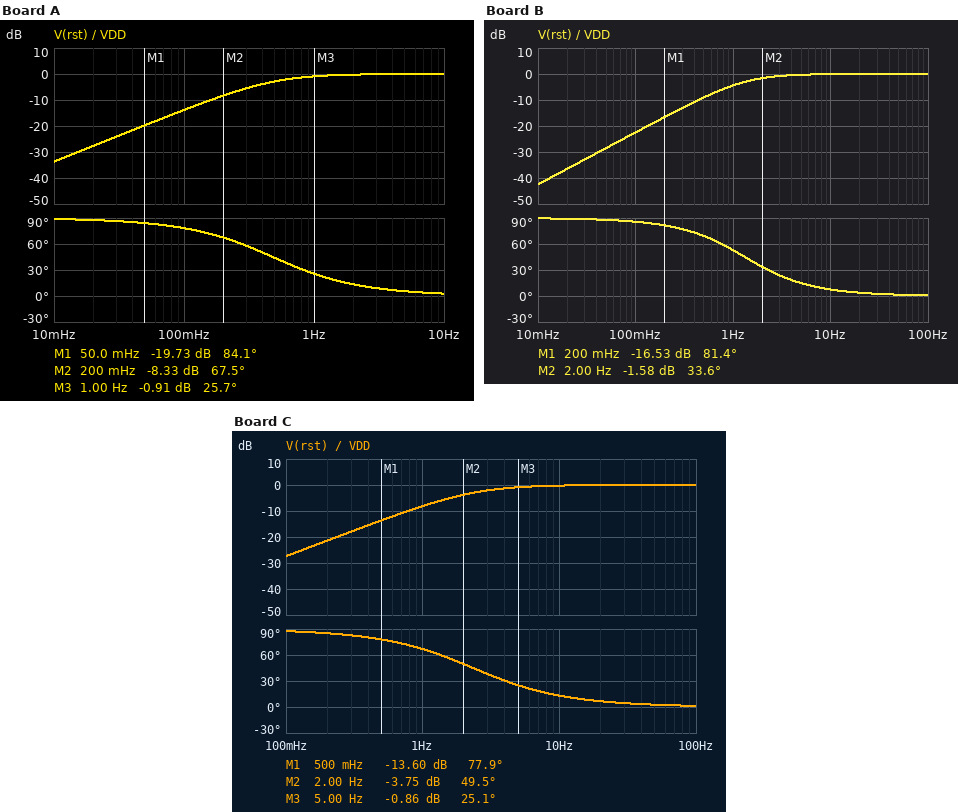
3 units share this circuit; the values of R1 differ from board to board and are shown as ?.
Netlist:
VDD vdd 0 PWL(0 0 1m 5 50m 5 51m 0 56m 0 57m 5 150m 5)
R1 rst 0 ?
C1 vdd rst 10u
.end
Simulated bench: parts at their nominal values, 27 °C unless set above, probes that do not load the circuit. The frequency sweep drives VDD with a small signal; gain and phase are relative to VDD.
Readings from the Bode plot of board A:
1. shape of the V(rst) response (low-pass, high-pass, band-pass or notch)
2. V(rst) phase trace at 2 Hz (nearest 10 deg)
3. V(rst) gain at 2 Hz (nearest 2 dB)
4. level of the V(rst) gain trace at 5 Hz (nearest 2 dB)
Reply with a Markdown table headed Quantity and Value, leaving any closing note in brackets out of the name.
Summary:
| Quantity | Value |
|---|---|
| shape of the V(rst) response | high-pass |
| V(rst) phase trace at 2 Hz | 10 deg |
| V(rst) gain at 2 Hz | 0 dB |
| level of the V(rst) gain trace at 5 Hz | 0 dB |
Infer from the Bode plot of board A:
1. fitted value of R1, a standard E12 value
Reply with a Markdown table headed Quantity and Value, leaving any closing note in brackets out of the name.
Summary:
| Quantity | Value |
|---|---|
| fitted value of R1, a standard E12 value | 33 kΩ |
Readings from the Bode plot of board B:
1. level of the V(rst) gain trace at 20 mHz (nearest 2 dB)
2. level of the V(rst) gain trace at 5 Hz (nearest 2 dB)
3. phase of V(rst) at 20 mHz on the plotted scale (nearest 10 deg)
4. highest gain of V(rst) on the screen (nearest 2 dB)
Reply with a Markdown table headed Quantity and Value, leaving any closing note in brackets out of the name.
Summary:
| Quantity | Value |
|---|---|
| level of the V(rst) gain trace at 20 mHz | -36 dB |
| level of the V(rst) gain trace at 5 Hz | 0 dB |
| phase of V(rst) at 20 mHz on the plotted scale | 90 deg |
| highest gain of V(rst) on the screen | 0 dB |
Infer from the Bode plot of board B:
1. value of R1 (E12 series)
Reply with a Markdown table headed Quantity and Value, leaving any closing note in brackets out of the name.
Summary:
| Quantity | Value |
|---|---|
| value of R1 | 12 kΩ |
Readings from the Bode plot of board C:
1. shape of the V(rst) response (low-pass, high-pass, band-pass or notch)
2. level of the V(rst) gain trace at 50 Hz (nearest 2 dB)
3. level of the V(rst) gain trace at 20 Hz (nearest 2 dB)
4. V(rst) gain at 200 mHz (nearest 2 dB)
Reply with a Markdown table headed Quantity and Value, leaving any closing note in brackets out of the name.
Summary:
| Quantity | Value |
|---|---|
| shape of the V(rst) response | high-pass |
| level of the V(rst) gain trace at 50 Hz | 0 dB |
| level of the V(rst) gain trace at 20 Hz | 0 dB |
| V(rst) gain at 200 mHz | -22 dB |
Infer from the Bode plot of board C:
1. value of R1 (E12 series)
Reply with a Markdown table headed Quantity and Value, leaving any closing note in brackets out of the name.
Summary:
| Quantity | Value |
|---|---|
| value of R1 | 6.8 kΩ |
